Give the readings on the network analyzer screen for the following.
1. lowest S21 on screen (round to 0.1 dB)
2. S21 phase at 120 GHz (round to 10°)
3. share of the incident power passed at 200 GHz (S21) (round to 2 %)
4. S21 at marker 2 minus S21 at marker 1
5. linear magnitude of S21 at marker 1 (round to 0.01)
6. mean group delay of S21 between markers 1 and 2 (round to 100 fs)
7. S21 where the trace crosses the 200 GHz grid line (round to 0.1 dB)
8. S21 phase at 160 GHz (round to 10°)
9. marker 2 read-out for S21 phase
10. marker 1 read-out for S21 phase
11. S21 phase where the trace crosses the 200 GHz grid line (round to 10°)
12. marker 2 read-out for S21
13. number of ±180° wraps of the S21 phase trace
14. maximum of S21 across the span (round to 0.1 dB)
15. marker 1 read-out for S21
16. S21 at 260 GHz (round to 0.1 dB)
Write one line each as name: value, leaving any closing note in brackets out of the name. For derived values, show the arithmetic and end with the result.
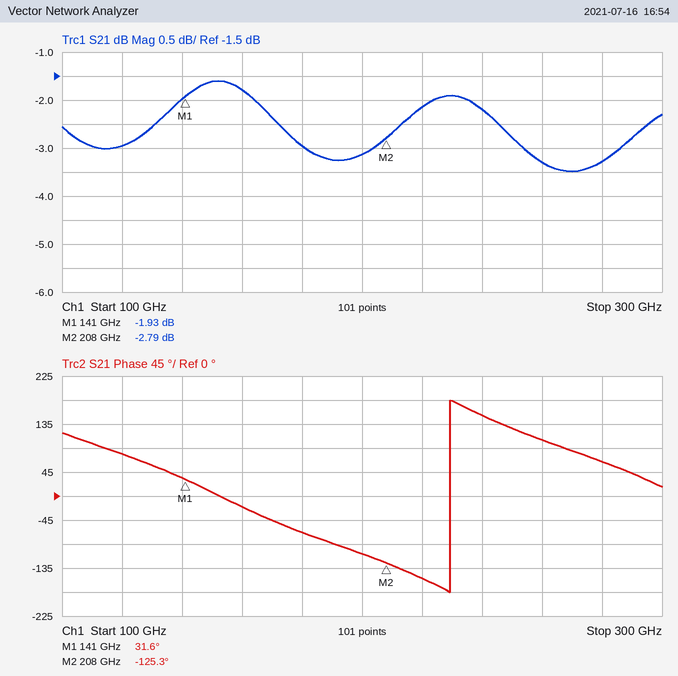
lowest S21 on screen: -3.5 dB
S21 phase at 120 GHz: 80°
share of the incident power passed at 200 GHz (S21): 10^(-3.1/10) ≈ 49.0 %, so 48 % to the nearest 2 %
S21 at marker 2 minus S21 at marker 1: -2.79 − (-1.93) = -0.86 dB
linear magnitude of S21 at marker 1: 10^(-1.93/20) ≈ 0.80
mean group delay of S21 between markers 1 and 2: −(-125.3° − (31.6°))/(360° × 67 GHz) ≈ 6.5 ps
S21 where the trace crosses the 200 GHz grid line: -3.1 dB
S21 phase at 160 GHz: -20°
marker 2 read-out for S21 phase: -125.3°
marker 1 read-out for S21 phase: 31.6°
S21 phase where the trace crosses the 200 GHz grid line: -110°
marker 2 read-out for S21: -2.79 dB
number of ±180° wraps of the S21 phase trace: 1
maximum of S21 across the span: -1.6 dB
marker 1 read-out for S21: -1.93 dB
S21 at 260 GHz: -3.3 dB
